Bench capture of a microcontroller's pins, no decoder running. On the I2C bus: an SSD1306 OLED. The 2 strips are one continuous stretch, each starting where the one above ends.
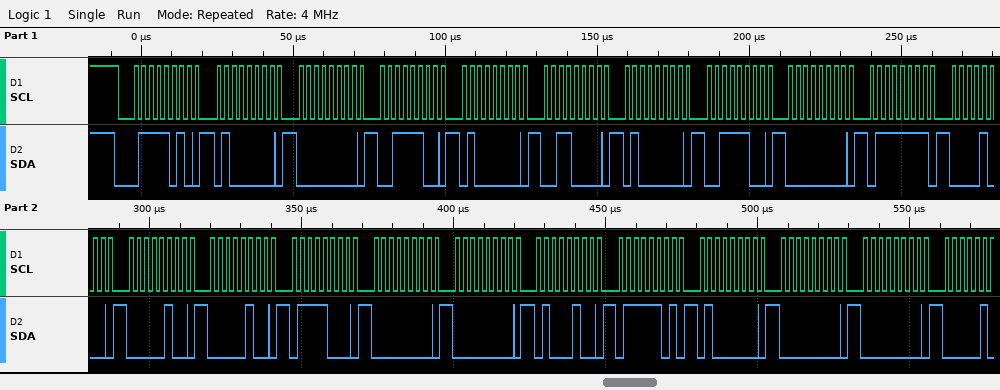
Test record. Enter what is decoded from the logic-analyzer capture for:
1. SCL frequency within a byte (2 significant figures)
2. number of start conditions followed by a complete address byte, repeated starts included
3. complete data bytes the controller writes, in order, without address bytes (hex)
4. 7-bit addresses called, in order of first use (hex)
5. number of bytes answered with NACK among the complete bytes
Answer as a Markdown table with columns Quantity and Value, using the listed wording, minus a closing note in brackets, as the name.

| Quantity | Value |
|---|---|
| SCL frequency within a byte | 400 kHz |
| number of start conditions followed by a complete address byte, repeated starts included | 1 |
| complete data bytes the controller writes, in order, without address bytes | 40 00 3C 40 30 40 3C 00 7F 08 04 04 78 00 00 44 7D 40 00 00 |
| 7-bit addresses called, in order of first use | 0x3D |
| number of bytes answered with NACK among the complete bytes | 0 |
